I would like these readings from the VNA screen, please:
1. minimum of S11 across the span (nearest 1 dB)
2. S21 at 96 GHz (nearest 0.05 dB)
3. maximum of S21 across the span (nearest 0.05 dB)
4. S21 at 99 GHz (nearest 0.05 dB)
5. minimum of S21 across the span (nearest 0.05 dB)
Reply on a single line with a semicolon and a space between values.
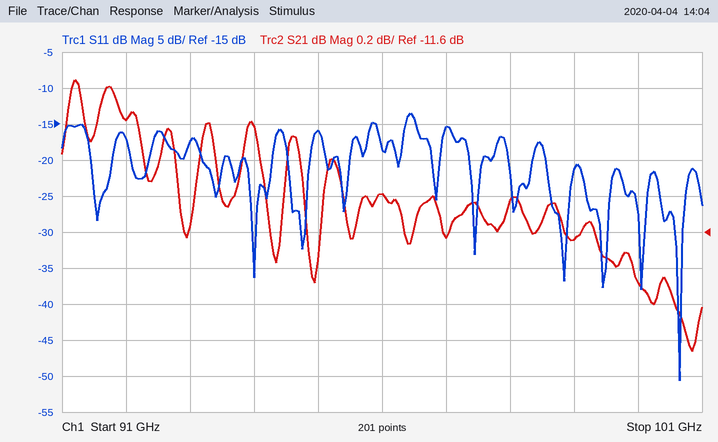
-51 dB; -11.40 dB; -10.75 dB; -11.65 dB; -12.25 dB
